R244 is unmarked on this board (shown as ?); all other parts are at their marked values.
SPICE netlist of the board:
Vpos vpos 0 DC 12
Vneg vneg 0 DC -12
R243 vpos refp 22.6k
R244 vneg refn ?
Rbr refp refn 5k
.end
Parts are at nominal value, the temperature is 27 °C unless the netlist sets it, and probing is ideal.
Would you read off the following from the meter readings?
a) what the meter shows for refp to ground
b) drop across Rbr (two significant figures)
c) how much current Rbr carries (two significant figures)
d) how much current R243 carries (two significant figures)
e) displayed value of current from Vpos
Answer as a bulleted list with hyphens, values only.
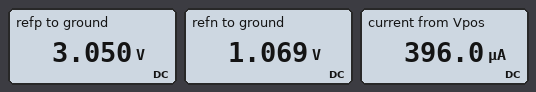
- 3.050 V
- 2.0 V
- 400 µA
- 400 µA
- 396.0 µA
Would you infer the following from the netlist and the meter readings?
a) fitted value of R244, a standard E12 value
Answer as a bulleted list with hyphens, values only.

- 33 kΩ
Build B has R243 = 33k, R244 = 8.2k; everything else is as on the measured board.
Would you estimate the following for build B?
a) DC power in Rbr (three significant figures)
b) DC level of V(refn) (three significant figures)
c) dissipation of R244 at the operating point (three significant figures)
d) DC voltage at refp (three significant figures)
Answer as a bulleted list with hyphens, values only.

- 1.35 mW
- -7.74 V
- 2.21 mW
- -5.14 V
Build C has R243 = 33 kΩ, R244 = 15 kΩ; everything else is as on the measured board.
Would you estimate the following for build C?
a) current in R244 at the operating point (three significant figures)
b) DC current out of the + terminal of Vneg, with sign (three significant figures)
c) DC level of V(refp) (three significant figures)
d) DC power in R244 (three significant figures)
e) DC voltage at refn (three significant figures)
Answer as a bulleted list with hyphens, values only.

- 453 µA
- -453 µA
- -2.94 V
- 3.08 mW
- -5.21 V
